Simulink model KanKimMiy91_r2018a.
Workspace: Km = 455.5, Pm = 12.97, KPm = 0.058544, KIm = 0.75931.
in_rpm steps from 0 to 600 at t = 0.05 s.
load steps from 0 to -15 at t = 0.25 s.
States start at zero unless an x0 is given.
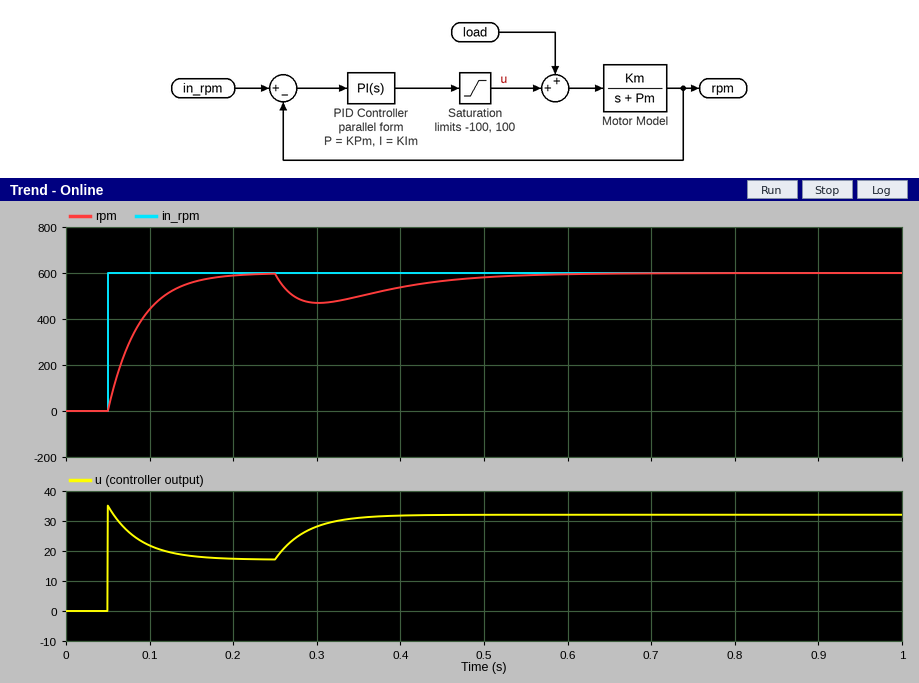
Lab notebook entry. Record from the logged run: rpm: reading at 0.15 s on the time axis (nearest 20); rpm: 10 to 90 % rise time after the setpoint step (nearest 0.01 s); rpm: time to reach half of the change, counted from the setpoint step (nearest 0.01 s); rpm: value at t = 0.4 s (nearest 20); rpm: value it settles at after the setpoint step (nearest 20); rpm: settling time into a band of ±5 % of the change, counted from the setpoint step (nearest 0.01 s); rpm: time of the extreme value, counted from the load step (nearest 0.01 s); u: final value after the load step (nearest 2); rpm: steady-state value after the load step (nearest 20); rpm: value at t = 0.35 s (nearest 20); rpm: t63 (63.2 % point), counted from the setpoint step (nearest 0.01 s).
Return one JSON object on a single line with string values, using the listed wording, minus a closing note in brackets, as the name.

{"rpm: reading at 0.15 s on the time axis": "560", "rpm: 10 to 90 % rise time after the setpoint step": "0.08 s", "rpm: time to reach half of the change, counted from the setpoint step": "0.03 s", "rpm: value at t = 0.4 s": "540", "rpm: value it settles at after the setpoint step": "600", "rpm: settling time into a band of ±5 % of the change, counted from the setpoint step": "0.11 s", "rpm: time of the extreme value, counted from the load step": "0.05 s", "u: final value after the load step": "32", "rpm: steady-state value after the load step": "600", "rpm: value at t = 0.35 s": "500", "rpm: t63 (63.2 % point), counted from the setpoint step": "0.04 s"}
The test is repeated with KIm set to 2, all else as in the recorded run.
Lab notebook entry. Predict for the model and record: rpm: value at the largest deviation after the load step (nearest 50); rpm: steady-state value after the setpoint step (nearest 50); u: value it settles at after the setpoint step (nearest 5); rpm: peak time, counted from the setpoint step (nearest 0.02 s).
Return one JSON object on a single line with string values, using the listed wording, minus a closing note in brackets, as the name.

{"rpm: value at the largest deviation after the load step": "500", "rpm: steady-state value after the setpoint step": "600", "u: value it settles at after the setpoint step": "15", "rpm: peak time, counted from the setpoint step": "0.10 s"}
